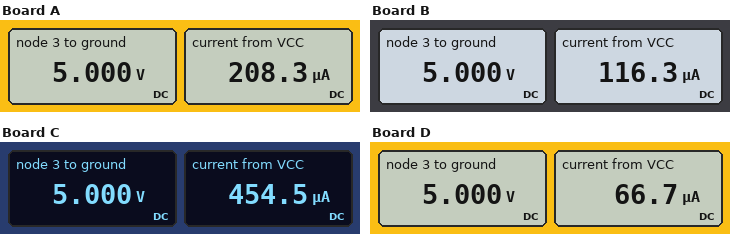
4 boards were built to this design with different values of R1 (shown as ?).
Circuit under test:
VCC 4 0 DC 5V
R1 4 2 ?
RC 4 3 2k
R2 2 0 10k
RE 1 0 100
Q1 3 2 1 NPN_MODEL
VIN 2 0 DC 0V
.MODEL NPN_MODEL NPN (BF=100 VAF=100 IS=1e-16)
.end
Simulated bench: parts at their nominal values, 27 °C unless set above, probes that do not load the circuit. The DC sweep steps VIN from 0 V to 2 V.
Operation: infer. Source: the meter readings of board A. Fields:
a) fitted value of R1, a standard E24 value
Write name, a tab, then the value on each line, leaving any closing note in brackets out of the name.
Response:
fitted value of R1, a standard E24 value	24 kΩ
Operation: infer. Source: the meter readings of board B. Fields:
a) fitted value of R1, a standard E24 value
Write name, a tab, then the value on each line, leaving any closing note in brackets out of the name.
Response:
fitted value of R1, a standard E24 value	43 kΩ
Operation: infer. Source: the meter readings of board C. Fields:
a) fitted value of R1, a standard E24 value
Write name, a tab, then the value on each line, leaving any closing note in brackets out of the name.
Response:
fitted value of R1, a standard E24 value	11 kΩ
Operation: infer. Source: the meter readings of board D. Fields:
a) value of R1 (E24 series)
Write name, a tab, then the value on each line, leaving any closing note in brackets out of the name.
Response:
value of R1	75 kΩ
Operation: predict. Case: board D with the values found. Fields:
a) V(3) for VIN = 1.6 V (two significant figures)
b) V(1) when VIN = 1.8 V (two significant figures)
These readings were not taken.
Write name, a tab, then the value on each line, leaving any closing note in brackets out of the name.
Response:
V(3) for VIN = 1.6 V	780 mV
V(1) when VIN = 1.8 V	950 mV
